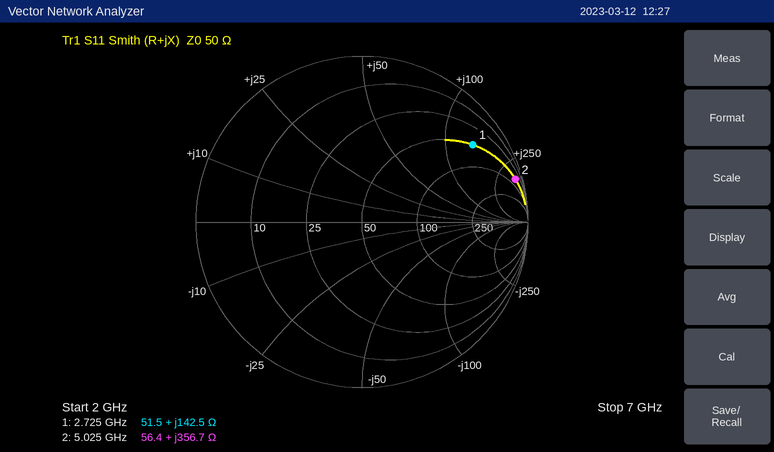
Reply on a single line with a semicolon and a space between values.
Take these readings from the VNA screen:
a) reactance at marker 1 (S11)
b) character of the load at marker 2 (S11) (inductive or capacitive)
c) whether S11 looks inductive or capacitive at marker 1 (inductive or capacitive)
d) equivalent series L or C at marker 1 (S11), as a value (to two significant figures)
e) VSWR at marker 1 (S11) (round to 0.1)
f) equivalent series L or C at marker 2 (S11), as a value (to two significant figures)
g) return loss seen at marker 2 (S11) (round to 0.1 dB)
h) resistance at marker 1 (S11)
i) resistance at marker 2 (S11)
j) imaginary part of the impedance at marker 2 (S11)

+142.5 Ω; inductive; inductive; 8.3 nH; 9.8; 11 nH; 0.4 dB; 51.5 Ω; 56.4 Ω; +356.7 Ω
